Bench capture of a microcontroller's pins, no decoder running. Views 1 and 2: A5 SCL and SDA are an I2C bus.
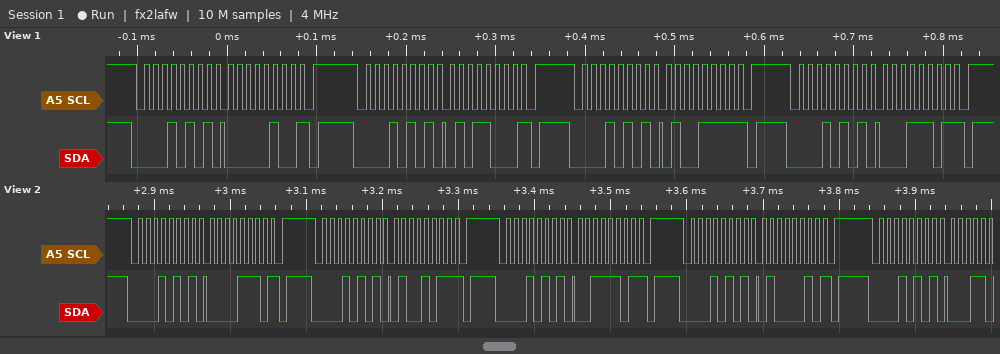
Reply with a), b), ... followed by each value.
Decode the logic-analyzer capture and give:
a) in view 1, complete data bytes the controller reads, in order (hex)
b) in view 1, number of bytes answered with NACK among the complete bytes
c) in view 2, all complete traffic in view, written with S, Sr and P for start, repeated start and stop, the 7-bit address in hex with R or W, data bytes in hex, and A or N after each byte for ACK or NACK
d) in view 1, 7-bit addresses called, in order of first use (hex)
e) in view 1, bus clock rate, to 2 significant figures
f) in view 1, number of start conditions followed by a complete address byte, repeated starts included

a) 04 58 4F 1D
b) 4
c) S 0AR A 0E N P S 0AR A 4B N P S 0AR A 3D N P S 0AR A 42 N P S 0AR A
d) 0x0A
e) 100 kHz
f) 4
